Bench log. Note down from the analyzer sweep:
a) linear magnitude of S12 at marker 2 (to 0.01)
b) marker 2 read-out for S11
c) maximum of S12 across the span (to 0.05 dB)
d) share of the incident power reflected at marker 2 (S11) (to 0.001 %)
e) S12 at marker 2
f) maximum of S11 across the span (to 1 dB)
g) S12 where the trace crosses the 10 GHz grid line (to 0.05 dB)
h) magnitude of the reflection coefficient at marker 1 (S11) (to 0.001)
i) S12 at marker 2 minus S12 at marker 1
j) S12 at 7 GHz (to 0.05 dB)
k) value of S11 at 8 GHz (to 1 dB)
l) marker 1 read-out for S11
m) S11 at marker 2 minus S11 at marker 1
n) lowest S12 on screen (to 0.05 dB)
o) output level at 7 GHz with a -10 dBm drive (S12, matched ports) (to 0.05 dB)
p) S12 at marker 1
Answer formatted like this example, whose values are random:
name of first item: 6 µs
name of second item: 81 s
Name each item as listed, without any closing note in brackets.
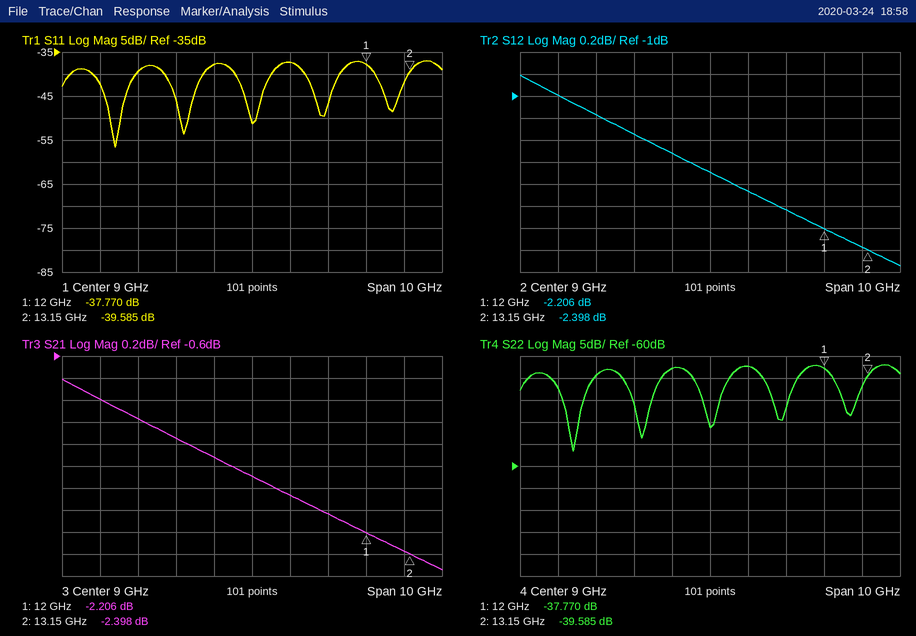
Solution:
linear magnitude of S12 at marker 2: 0.76
marker 2 read-out for S11: -39.585 dB
maximum of S12 across the span: -0.80 dB
share of the incident power reflected at marker 2 (S11): 0.011 %
S12 at marker 2: -2.398 dB
maximum of S11 across the span: -37 dB
S12 where the trace crosses the 10 GHz grid line: -1.85 dB
magnitude of the reflection coefficient at marker 1 (S11): 0.013
S12 at marker 2 minus S12 at marker 1: -0.192 dB
S12 at 7 GHz: -1.35 dB
value of S11 at 8 GHz: -38 dB
marker 1 read-out for S11: -37.770 dB
S11 at marker 2 minus S11 at marker 1: -1.815 dB
lowest S12 on screen: -2.55 dB
output level at 7 GHz with a -10 dBm drive (S12, matched ports): -11.35 dBm
S12 at marker 1: -2.206 dB
